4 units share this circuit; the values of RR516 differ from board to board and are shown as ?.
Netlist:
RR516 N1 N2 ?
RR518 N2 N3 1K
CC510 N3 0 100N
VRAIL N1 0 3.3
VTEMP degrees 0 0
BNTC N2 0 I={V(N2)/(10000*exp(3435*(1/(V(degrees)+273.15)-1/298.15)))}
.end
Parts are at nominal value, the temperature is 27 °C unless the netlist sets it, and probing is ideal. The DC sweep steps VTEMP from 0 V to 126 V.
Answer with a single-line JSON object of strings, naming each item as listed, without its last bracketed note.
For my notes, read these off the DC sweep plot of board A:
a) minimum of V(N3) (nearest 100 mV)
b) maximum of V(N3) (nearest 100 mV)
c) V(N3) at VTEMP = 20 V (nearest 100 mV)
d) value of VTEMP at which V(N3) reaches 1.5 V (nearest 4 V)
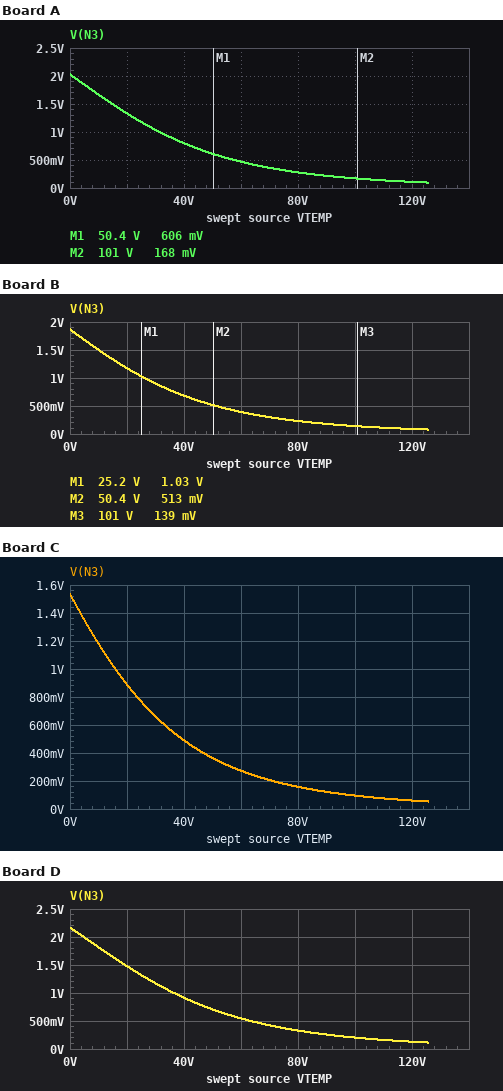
{"minimum of V(N3)": "100 mV", "maximum of V(N3)": "2.0 V", "V(N3) at VTEMP = 20 V": "1.3 V", "value of VTEMP at which V(N3) reaches 1.5 V": "16 V"}
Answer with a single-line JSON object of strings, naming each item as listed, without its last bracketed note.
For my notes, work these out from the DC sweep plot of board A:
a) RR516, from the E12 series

{"RR516, from the E12 series": "18 kΩ"}
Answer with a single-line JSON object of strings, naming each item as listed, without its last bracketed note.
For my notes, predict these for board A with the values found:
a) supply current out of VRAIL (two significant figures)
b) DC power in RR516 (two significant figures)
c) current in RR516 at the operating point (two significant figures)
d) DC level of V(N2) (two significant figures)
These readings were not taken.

{"supply current out of VRAIL": "71 µA", "DC power in RR516": "90 µW", "current in RR516 at the operating point": "71 µA", "DC level of V(N2)": "2.0 V"}
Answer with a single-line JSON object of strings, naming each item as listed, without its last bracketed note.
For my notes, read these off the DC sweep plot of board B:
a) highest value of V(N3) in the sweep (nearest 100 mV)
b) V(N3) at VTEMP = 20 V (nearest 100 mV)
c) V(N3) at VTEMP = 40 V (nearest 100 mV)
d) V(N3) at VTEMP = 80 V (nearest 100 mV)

{"highest value of V(N3) in the sweep": "1.9 V", "V(N3) at VTEMP = 20 V": "1.2 V", "V(N3) at VTEMP = 40 V": "700 mV", "V(N3) at VTEMP = 80 V": "200 mV"}
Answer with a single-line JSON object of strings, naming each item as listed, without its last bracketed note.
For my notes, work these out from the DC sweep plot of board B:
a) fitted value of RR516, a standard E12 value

{"fitted value of RR516, a standard E12 value": "22 kΩ"}
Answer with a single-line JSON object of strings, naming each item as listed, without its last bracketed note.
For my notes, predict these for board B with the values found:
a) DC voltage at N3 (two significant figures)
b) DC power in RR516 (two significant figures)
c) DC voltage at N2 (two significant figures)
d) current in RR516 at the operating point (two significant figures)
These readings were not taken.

{"DC voltage at N3": "1.9 V", "DC power in RR516": "93 µW", "DC voltage at N2": "1.9 V", "current in RR516 at the operating point": "65 µA"}
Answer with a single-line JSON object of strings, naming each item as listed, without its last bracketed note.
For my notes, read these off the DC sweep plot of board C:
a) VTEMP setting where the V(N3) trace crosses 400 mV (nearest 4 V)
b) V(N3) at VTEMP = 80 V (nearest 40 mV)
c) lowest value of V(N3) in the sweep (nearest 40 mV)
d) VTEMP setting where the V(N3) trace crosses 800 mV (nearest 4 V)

{"VTEMP setting where the V(N3) trace crosses 400 mV": "48 V", "V(N3) at VTEMP = 80 V": "160 mV", "lowest value of V(N3) in the sweep": "40 mV", "VTEMP setting where the V(N3) trace crosses 800 mV": "24 V"}
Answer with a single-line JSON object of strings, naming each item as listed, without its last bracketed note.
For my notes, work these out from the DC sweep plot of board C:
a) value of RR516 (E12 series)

{"value of RR516": "33 kΩ"}
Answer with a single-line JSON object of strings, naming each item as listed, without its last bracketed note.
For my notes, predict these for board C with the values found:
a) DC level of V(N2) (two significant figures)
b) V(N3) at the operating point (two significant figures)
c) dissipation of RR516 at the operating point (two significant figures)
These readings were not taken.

{"DC level of V(N2)": "1.5 V", "V(N3) at the operating point": "1.5 V", "dissipation of RR516 at the operating point": "94 µW"}
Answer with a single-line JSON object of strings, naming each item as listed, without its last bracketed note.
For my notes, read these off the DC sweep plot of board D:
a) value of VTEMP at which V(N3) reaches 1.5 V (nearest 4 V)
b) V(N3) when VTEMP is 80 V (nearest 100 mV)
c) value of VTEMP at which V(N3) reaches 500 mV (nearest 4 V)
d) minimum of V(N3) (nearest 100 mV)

{"value of VTEMP at which V(N3) reaches 1.5 V": "20 V", "V(N3) when VTEMP is 80 V": "300 mV", "value of VTEMP at which V(N3) reaches 500 mV": "64 V", "minimum of V(N3)": "100 mV"}
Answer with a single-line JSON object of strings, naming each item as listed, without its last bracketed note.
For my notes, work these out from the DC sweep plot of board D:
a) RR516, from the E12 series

{"RR516, from the E12 series": "15 kΩ"}
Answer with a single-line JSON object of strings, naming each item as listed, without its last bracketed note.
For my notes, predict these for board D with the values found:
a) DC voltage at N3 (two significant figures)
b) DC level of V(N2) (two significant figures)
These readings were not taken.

{"DC voltage at N3": "2.2 V", "DC level of V(N2)": "2.2 V"}
